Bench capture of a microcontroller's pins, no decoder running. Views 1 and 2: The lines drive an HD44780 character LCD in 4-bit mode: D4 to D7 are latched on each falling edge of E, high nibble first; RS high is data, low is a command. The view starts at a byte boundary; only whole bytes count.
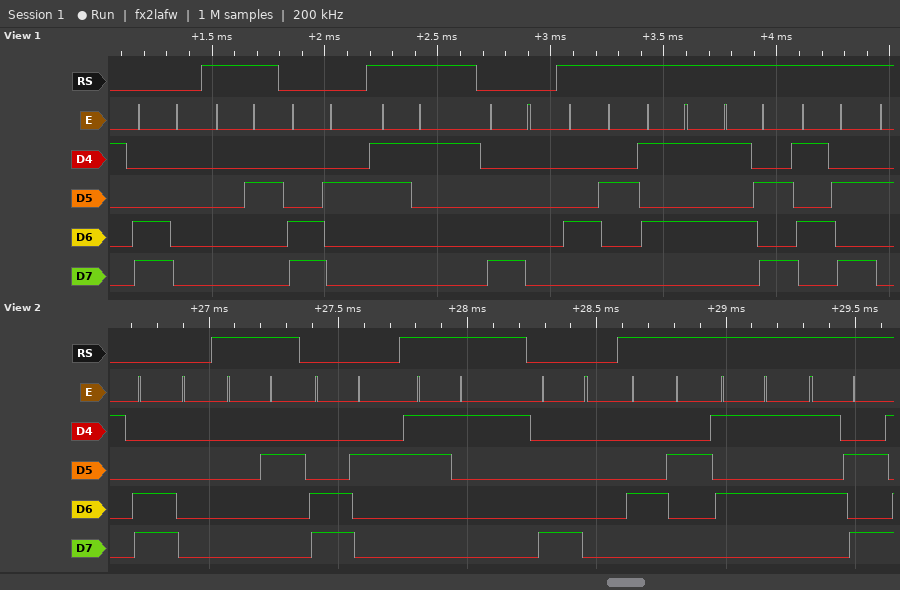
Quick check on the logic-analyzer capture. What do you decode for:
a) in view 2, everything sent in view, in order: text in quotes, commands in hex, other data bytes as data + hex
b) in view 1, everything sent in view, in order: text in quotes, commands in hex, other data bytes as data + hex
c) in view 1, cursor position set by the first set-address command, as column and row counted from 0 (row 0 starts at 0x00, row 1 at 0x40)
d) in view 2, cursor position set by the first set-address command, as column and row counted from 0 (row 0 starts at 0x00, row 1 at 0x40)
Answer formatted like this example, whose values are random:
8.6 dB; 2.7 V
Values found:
0xC0 data 02 0xC2 "1" 0x80 "BUZ"; 0xC0 data 02 0xC2 "1" 0x80 "BUZZ"; column 0, row 1; column 0, row 1
